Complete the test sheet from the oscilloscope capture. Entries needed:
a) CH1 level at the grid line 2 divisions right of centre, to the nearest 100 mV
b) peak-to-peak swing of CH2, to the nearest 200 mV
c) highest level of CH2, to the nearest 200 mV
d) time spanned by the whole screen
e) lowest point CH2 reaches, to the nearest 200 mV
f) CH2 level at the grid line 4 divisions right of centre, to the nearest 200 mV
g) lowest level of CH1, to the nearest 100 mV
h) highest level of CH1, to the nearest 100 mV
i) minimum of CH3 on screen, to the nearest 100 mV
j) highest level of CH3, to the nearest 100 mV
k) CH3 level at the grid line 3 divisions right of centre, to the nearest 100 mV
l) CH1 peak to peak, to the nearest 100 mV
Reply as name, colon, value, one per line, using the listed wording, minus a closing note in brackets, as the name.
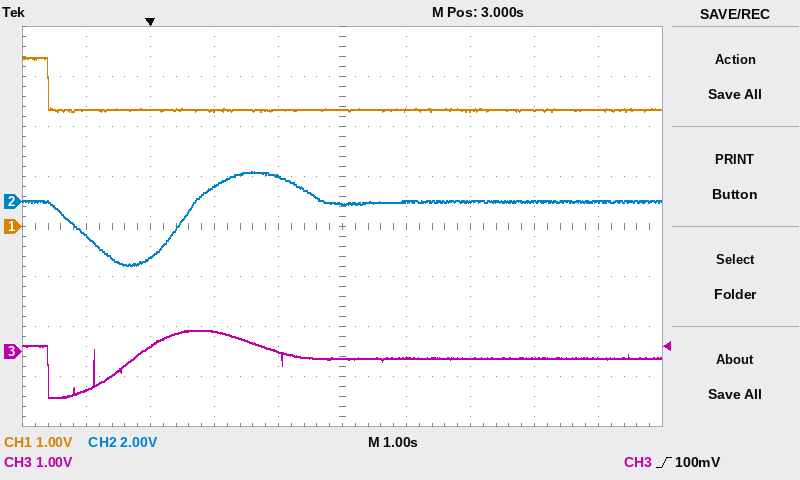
CH1 level at the grid line 2 divisions right of centre, to the nearest 100 mV: 2.3 V
peak-to-peak swing of CH2, to the nearest 200 mV: 3.8 V
highest level of CH2, to the nearest 200 mV: 1.2 V
time spanned by the whole screen: 10 s
lowest point CH2 reaches, to the nearest 200 mV: -2.6 V
CH2 level at the grid line 4 divisions right of centre, to the nearest 200 mV: 0.0 V
lowest level of CH1, to the nearest 100 mV: 2.3 V
highest level of CH1, to the nearest 100 mV: 3.4 V
minimum of CH3 on screen, to the nearest 100 mV: -900 mV
highest level of CH3, to the nearest 100 mV: 400 mV
CH3 level at the grid line 3 divisions right of centre, to the nearest 100 mV: -100 mV
CH1 peak to peak, to the nearest 100 mV: 1.1 V
